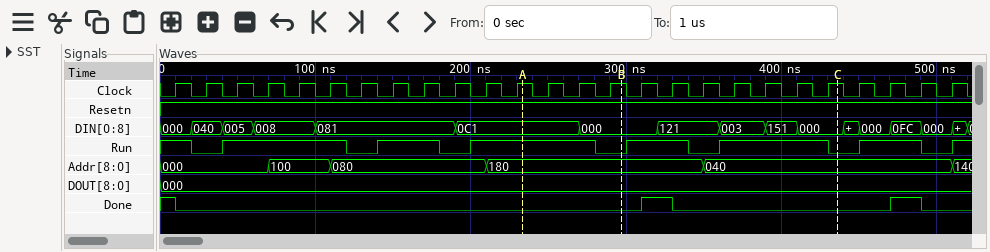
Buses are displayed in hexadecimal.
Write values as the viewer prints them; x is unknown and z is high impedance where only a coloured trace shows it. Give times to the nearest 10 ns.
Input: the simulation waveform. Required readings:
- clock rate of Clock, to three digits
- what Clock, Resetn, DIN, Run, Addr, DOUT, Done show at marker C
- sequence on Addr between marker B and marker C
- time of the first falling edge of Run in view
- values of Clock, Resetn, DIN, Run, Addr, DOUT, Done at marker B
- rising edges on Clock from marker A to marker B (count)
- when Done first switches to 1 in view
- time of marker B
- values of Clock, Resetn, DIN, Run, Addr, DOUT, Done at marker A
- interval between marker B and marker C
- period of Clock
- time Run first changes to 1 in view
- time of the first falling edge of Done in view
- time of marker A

50.0 MHz
Clock=1, Resetn=1, DIN=000, Run=0, Addr=040, DOUT=000, Done=0
180, 040
20 ns
Clock=1, Resetn=1, DIN=000, Run=0, Addr=180, DOUT=000, Done=0
3
310 ns
300 ns
Clock=1, Resetn=1, DIN=0C1, Run=1, Addr=180, DOUT=000, Done=0
140 ns
20 ns
40 ns
10 ns
230 ns
